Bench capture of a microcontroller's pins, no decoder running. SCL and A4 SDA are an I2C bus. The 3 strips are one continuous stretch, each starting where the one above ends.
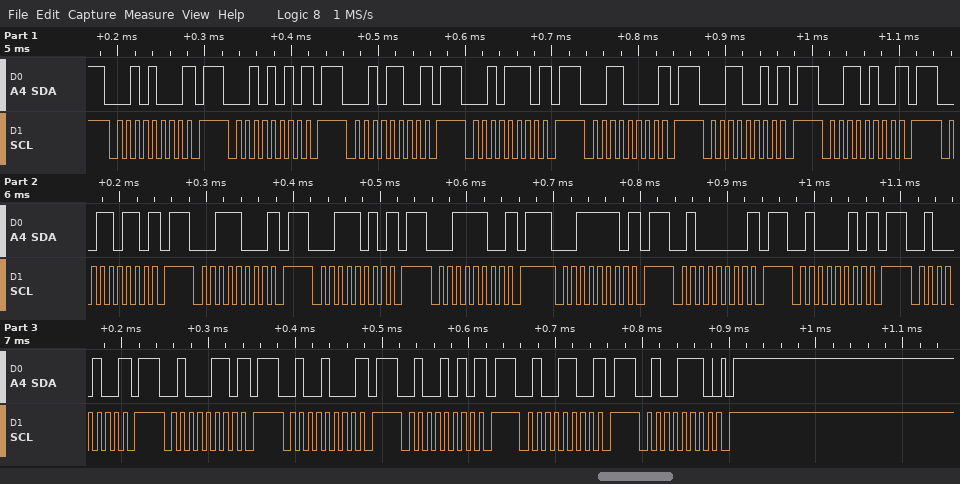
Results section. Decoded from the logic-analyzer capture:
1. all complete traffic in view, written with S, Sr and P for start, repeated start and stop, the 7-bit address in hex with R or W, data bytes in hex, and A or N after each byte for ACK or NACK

S 14W N P S 15W N P S 16W N P S 17W N P S 18W N P S 19W N P S 1AW N P S 1BW N P S 1CW N P S 1DW N P S 1EW N P S 1FW N P S 20W N P S 21W N P S 22W N P S 23W N P S 24W N P S 25W N P S 26W N P S 27W A P
